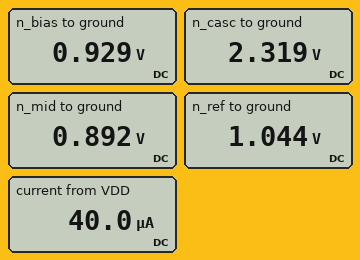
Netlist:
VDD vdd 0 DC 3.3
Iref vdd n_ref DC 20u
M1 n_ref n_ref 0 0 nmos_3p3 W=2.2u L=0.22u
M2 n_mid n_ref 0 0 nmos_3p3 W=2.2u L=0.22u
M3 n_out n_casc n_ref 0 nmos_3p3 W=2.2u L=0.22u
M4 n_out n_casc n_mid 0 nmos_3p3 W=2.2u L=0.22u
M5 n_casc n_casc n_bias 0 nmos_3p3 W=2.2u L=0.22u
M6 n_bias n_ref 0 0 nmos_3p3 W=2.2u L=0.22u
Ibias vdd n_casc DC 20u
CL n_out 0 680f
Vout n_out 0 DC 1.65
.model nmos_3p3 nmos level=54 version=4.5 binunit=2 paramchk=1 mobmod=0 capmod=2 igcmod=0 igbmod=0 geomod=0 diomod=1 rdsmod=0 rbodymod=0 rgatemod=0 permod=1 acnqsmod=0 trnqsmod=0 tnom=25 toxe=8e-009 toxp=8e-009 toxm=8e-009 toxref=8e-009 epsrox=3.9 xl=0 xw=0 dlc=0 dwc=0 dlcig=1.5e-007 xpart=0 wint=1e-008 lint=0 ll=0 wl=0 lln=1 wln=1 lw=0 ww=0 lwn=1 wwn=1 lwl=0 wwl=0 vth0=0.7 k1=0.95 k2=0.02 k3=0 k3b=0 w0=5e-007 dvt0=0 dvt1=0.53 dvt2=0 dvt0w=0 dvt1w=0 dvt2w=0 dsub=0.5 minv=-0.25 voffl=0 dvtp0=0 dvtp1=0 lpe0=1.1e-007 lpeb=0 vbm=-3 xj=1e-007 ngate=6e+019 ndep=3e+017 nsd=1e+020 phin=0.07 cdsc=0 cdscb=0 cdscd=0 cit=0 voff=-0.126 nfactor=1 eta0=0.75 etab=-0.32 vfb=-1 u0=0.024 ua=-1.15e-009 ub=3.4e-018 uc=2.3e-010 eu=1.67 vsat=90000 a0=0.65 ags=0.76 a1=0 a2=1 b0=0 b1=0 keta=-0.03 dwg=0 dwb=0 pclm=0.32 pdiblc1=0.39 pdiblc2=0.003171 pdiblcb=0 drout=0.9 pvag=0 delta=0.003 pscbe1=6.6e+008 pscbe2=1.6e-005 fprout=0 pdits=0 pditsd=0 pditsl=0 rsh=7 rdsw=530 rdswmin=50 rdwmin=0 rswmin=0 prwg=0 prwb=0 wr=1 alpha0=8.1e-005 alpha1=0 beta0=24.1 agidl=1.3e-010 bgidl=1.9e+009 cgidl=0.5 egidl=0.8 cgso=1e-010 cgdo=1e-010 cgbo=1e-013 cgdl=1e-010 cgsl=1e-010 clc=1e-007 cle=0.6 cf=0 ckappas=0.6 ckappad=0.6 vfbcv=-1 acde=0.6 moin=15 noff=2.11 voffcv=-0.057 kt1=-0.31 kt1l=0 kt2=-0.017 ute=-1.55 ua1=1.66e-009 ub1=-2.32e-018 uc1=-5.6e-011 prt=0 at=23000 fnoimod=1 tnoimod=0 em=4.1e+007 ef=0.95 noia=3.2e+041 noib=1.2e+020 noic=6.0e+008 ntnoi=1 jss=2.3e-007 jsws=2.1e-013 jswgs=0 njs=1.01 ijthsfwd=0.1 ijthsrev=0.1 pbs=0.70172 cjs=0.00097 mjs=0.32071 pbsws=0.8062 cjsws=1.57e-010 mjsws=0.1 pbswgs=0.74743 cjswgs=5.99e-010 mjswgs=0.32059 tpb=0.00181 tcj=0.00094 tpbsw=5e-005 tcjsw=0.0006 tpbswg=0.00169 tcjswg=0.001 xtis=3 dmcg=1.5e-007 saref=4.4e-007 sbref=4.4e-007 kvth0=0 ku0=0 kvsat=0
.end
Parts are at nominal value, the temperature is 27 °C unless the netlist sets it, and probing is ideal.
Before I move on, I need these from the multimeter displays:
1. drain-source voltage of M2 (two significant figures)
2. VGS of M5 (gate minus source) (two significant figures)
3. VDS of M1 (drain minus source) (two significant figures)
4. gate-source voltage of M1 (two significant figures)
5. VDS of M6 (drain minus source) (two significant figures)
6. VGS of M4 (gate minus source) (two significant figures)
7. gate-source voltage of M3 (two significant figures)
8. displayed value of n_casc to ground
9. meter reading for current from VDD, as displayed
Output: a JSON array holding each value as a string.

["890 mV", "1.4 V", "1.0 V", "1.0 V", "930 mV", "1.4 V", "1.3 V", "2.319 V", "40.0 µA"]
